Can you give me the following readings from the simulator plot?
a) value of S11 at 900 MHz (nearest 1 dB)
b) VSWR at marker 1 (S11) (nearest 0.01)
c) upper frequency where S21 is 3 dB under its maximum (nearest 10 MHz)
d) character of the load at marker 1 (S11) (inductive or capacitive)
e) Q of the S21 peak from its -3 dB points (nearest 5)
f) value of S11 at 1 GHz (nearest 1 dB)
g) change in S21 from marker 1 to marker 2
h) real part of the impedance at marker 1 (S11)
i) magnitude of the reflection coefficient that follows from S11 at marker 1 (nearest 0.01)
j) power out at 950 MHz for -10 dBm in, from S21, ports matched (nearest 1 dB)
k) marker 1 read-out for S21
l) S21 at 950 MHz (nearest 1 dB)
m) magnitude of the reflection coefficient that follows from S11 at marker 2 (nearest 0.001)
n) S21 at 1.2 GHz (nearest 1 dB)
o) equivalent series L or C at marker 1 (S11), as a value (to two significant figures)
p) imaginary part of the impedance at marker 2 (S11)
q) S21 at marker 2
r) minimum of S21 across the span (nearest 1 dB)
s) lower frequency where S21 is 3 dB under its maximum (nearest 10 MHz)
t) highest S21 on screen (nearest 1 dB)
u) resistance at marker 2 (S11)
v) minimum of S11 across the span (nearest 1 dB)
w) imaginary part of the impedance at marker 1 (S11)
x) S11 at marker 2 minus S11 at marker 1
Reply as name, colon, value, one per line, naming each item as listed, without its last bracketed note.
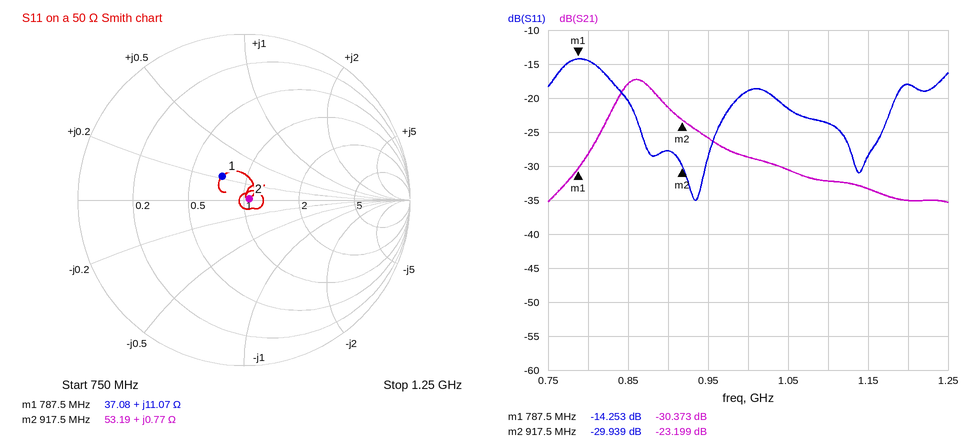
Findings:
value of S11 at 900 MHz: -28 dB
VSWR at marker 1 (S11): 1.48
upper frequency where S21 is 3 dB under its maximum: 890 MHz
character of the load at marker 1 (S11): inductive
Q of the S21 peak from its -3 dB points: 15
value of S11 at 1 GHz: -19 dB
change in S21 from marker 1 to marker 2: 7.174 dB
real part of the impedance at marker 1: 37.08 Ω
magnitude of the reflection coefficient that follows from S11 at marker 1: 0.19
power out at 950 MHz for -10 dBm in, from S21, ports matched: -36 dBm
marker 1 read-out for S21: -30.373 dB
S21 at 950 MHz: -26 dB
magnitude of the reflection coefficient that follows from S11 at marker 2: 0.032
S21 at 1.2 GHz: -35 dB
equivalent series L or C at marker 1 (S11), as a value: 2.2 nH
imaginary part of the impedance at marker 2: +0.77 Ω
S21 at marker 2: -23.199 dB
minimum of S21 across the span: -35 dB
lower frequency where S21 is 3 dB under its maximum: 840 MHz
highest S21 on screen: -17 dB
resistance at marker 2: 53.19 Ω
minimum of S11 across the span: -35 dB
imaginary part of the impedance at marker 1: +11.07 Ω
S11 at marker 2 minus S11 at marker 1: -15.686 dB
